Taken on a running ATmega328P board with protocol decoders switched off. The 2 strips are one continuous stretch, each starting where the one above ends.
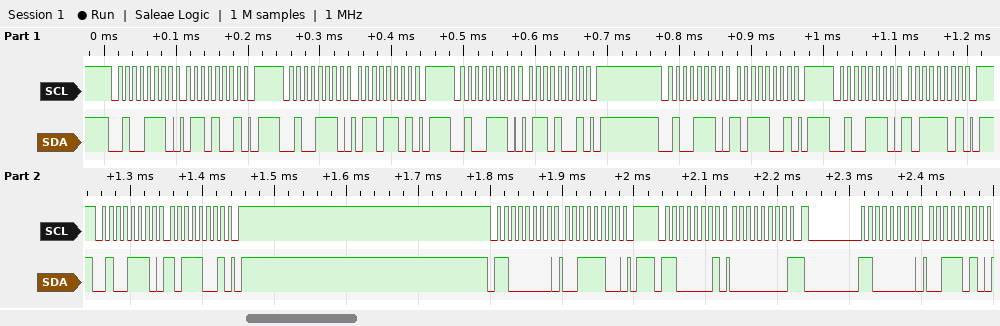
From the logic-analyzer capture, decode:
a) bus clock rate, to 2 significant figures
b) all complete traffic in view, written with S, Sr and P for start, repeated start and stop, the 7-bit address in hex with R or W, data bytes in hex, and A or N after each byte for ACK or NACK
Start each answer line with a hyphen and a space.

- 100 kHz
- S 27W A 69 A P S 27W A 6D A P S 27W A 69 A P S 27W A B9 A P S 27W A BD A P S 27W A B9 A P S 60W A 3C A P S 60R A 00 N Sr 60W A 3A A
